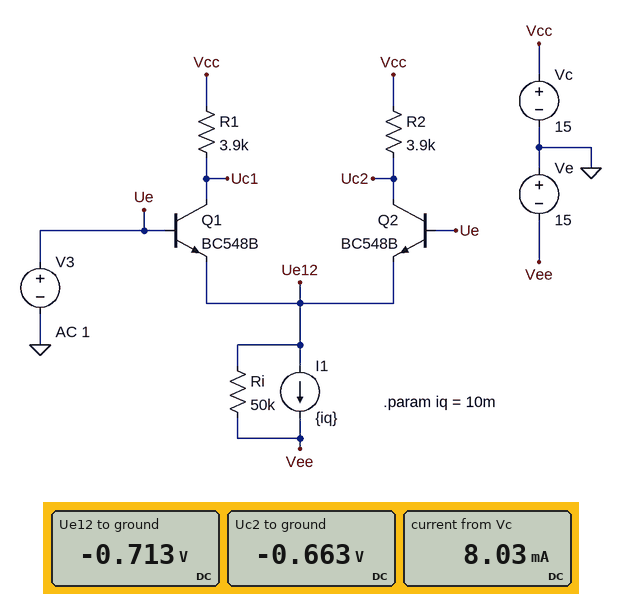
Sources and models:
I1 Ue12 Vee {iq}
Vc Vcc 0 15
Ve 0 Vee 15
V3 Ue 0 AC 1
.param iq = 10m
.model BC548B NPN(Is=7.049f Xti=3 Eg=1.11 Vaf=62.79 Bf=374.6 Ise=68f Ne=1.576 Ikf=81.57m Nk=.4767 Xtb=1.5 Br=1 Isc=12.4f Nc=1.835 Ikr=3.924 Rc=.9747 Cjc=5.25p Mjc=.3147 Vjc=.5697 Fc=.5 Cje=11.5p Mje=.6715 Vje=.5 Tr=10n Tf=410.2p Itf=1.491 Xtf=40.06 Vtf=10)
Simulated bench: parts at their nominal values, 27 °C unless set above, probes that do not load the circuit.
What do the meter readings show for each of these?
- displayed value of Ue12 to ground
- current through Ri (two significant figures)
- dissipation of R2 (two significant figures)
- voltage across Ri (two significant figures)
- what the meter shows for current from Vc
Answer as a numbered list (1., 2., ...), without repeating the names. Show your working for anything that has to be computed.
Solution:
1. -0.713 V
2. (-713 mV - (-15 V)) / 50 kΩ = 290 µA
3. (15 V - (-663 mV))^2 / 3.9 kΩ = 63 mW
4. -713 mV - (-15 V) = 14 V
5. 8.03 mA
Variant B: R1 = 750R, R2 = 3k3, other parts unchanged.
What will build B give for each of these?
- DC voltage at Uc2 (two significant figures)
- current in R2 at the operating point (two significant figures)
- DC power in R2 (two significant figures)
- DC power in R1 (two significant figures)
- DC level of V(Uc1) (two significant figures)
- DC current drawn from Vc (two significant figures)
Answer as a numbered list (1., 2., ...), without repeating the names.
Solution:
1. -500 mV
2. 4.7 mA
3. 73 mW
4. 23 mW
5. 11 V
6. 10 mA
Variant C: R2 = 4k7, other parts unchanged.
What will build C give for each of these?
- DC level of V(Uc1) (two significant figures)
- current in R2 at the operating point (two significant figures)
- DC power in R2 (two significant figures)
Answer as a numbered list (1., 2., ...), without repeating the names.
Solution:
1. -670 mV
2. 3.3 mA
3. 52 mW
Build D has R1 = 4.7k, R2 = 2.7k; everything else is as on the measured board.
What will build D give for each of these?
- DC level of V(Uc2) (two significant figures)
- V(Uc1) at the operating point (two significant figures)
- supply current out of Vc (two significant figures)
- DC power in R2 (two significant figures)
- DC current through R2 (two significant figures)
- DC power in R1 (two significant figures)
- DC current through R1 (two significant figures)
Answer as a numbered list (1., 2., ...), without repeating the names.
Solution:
1. -390 mV
2. -670 mV
3. 9.0 mA
4. 88 mW
5. 5.7 mA
6. 52 mW
7. 3.3 mA
